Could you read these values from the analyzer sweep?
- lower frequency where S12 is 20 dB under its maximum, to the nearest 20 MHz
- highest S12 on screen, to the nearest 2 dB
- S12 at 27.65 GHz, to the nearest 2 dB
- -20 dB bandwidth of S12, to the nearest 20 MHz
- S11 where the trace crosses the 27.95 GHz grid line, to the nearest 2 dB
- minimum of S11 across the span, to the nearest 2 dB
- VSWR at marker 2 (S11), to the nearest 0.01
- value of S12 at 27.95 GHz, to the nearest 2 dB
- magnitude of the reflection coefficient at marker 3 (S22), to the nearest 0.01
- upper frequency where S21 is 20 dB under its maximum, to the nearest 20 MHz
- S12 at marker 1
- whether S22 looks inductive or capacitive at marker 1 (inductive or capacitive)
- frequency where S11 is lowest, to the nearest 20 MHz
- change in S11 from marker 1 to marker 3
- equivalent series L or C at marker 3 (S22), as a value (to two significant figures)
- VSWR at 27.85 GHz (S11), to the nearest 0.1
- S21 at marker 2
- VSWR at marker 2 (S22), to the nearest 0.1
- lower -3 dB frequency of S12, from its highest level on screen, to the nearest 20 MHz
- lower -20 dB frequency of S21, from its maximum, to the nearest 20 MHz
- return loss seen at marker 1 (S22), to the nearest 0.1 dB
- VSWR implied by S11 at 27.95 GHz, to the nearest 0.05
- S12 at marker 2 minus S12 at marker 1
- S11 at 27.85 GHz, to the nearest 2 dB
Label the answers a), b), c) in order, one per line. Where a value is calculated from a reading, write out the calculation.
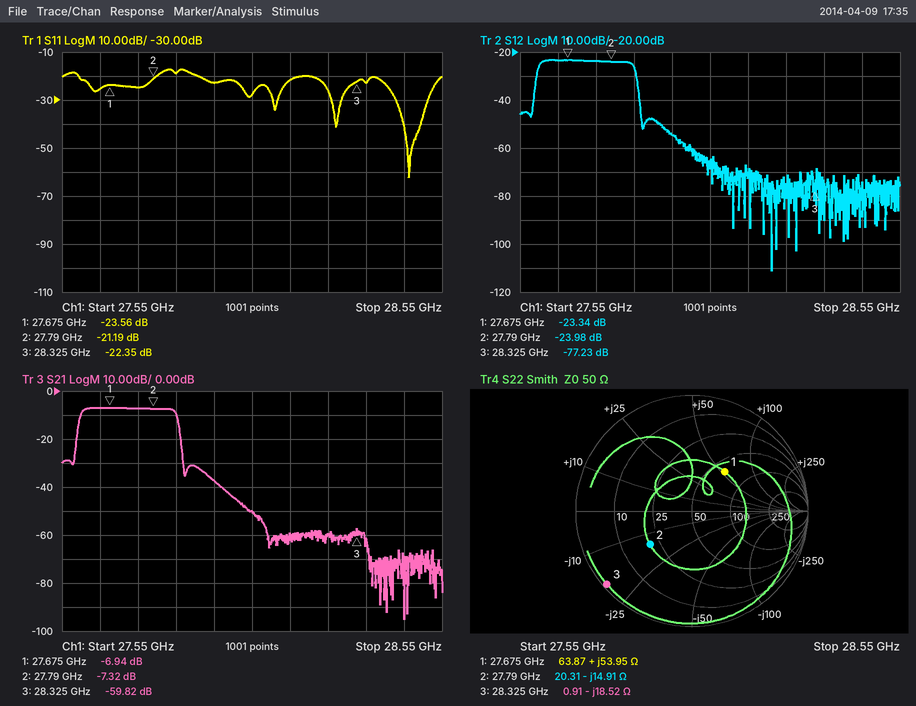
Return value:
a) 27.58 GHz
b) -24 dB
c) -24 dB
d) 27.86 GHz − 27.58 GHz = 280 MHz
e) -22 dB
f) -62 dB
g) (1 + 0.0872)/(1 − 0.0872) ≈ 1.19
h) -54 dB
i) 0.97
j) 27.86 GHz
k) -23.34 dB
l) inductive
m) 28.46 GHz
n) -22.35 − (-23.56) = 1.21 dB
o) C = 1/(2π × 28.325 GHz × 18.52 Ω) ≈ 303 fF, so 300 fF to two significant figures
p) |Γ| = 10^(-18/20) = 0.1259; VSWR = (1 + 0.1259)/(1 − 0.1259) ≈ 1.3
q) -7.32 dB
r) 2.7
s) 27.60 GHz
t) 27.58 GHz
u) 7.1 dB
v) |Γ| = 10^(-22/20) = 0.0794; VSWR = (1 + 0.0794)/(1 − 0.0794) ≈ 1.17, so 1.15 to the nearest 0.05
w) -23.98 − (-23.34) = -0.64 dB
x) -18 dB
